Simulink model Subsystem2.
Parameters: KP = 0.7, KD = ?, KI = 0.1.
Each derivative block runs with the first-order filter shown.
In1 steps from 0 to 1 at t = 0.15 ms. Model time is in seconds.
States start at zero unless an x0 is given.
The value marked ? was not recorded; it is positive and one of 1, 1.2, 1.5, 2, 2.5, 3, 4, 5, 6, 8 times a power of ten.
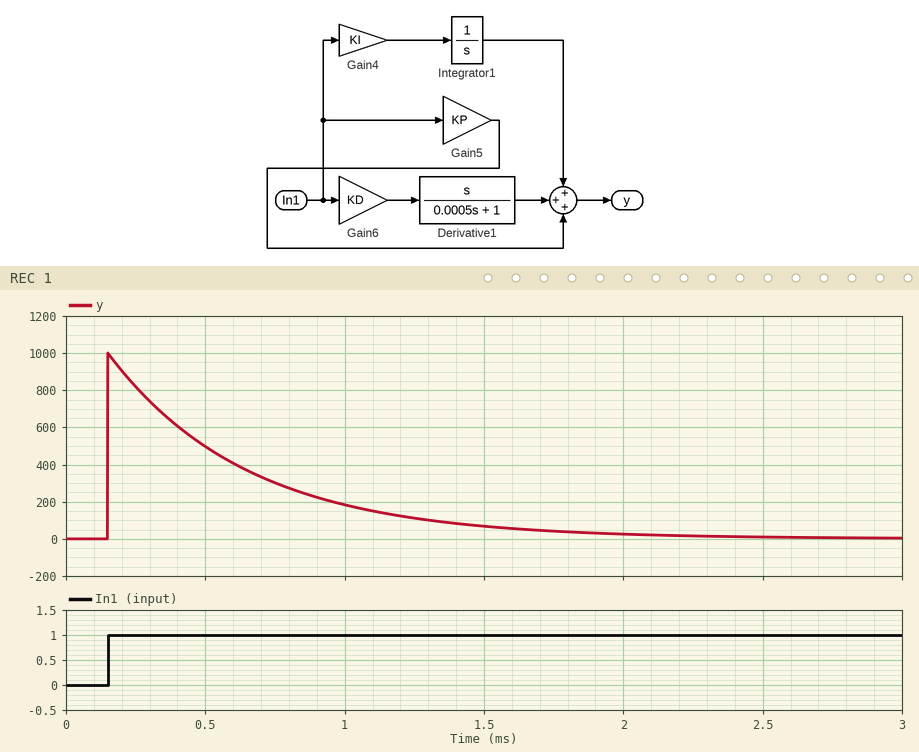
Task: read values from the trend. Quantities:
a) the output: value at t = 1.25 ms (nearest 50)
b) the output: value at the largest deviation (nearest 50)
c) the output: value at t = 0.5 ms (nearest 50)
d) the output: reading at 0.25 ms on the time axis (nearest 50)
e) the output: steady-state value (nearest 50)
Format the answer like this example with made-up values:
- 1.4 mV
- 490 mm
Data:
- 100
- 1000
- 500
- 800
- 0
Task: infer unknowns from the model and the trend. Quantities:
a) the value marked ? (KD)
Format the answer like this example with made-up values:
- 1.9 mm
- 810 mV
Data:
- 0.5
